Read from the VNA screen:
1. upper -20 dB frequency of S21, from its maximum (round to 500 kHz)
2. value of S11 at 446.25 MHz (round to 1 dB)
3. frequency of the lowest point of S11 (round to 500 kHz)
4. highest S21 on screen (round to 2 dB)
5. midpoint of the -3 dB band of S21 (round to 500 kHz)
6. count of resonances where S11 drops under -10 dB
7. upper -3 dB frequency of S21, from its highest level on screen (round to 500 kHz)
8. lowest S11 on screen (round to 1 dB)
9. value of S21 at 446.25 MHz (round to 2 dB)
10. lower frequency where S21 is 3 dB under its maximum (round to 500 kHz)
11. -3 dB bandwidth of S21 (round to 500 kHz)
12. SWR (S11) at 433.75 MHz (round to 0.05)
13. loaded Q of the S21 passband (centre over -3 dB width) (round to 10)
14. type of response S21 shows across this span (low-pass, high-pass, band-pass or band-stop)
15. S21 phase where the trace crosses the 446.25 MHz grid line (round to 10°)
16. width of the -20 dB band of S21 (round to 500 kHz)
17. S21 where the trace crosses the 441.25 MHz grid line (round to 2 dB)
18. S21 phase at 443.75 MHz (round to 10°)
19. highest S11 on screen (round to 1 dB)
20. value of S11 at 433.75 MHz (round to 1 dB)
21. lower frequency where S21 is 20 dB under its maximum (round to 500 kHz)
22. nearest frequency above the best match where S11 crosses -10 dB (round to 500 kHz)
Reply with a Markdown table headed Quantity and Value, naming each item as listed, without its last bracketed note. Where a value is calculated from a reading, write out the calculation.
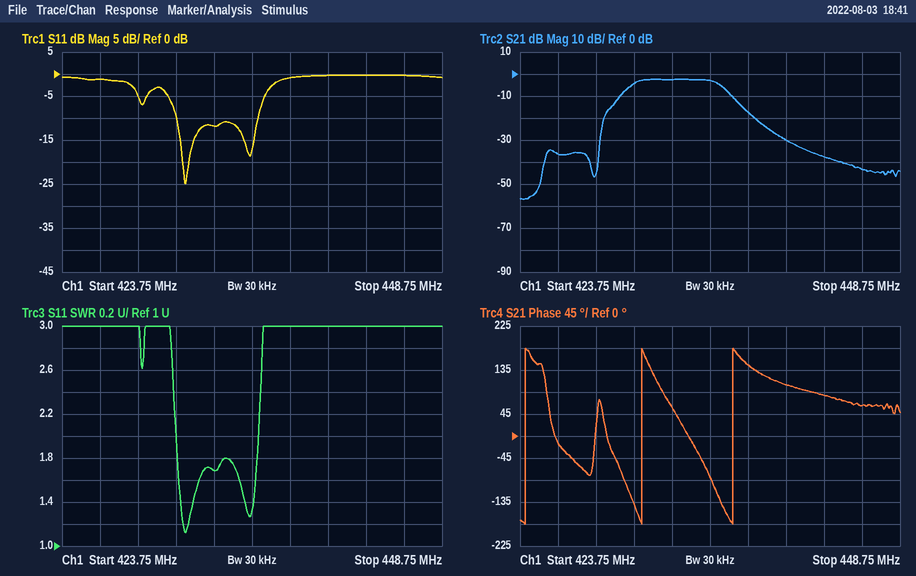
| Quantity | Value |
|---|---|
| upper -20 dB frequency of S21, from its maximum | 439.5 MHz |
| value of S11 at 446.25 MHz | 0 dB |
| frequency of the lowest point of S11 | 432.0 MHz |
| highest S21 on screen | -2 dB |
| midpoint of the -3 dB band of S21 | 434.0 MHz |
| count of resonances where S11 drops under -10 dB | 2 |
| upper -3 dB frequency of S21, from its highest level on screen | 437.0 MHz |
| lowest S11 on screen | -25 dB |
| value of S21 at 446.25 MHz | -44 dB |
| lower frequency where S21 is 3 dB under its maximum | 431.0 MHz |
| -3 dB bandwidth of S21 | 437.0 MHz − 431.0 MHz = 6.0 MHz |
| SWR (S11) at 433.75 MHz | 1.70 |
| loaded Q of the S21 passband (centre over -3 dB width) | 434 MHz / 6 MHz ≈ 72.3, so 70 to the nearest 10 |
| type of response S21 shows across this span | band-pass |
| S21 phase where the trace crosses the 446.25 MHz grid line | 60° |
| width of the -20 dB band of S21 | 439.5 MHz − 429.0 MHz = 10.5 MHz |
| S21 where the trace crosses the 441.25 MHz grid line | -30 dB |
| S21 phase at 443.75 MHz | 80° |
| highest S11 on screen | 0 dB |
| value of S11 at 433.75 MHz | -12 dB |
| lower frequency where S21 is 20 dB under its maximum | 429.0 MHz |
| nearest frequency above the best match where S11 crosses -10 dB | 436.5 MHz |
